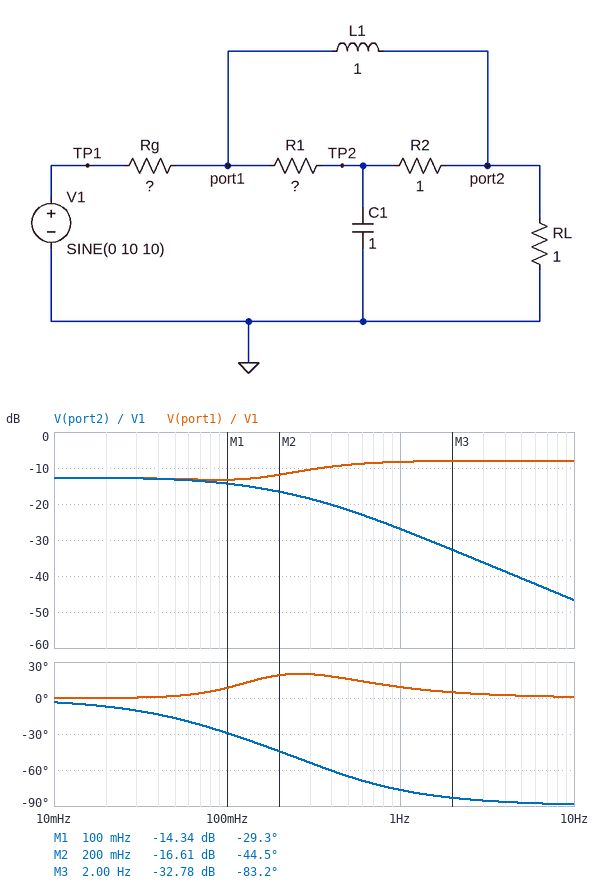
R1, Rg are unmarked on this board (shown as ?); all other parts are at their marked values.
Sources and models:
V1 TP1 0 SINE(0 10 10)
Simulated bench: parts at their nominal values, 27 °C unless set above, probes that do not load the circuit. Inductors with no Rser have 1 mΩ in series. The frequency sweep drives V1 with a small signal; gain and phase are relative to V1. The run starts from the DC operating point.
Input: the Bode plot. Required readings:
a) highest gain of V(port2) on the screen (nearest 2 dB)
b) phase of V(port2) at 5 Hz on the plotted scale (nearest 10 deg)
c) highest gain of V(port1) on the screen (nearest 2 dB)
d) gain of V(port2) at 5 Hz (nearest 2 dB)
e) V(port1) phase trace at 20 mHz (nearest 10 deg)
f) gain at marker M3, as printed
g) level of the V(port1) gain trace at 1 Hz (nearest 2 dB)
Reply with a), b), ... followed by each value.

a) -12 dB
b) -90 deg
c) -8 dB
d) -40 dB
e) 0 deg
f) -32.78 dB
g) -8 dB
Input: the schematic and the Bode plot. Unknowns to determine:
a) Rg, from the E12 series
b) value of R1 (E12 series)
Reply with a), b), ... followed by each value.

a) 3.3 Ω
b) 2.2 Ω
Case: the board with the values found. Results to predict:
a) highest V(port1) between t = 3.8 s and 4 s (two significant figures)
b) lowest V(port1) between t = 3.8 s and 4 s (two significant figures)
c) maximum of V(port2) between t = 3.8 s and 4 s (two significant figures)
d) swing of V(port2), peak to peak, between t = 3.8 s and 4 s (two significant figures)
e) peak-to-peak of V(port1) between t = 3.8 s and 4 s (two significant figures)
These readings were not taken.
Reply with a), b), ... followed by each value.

a) 4.0 V
b) -4.0 V
c) 47 mV
d) 93 mV
e) 8.0 V
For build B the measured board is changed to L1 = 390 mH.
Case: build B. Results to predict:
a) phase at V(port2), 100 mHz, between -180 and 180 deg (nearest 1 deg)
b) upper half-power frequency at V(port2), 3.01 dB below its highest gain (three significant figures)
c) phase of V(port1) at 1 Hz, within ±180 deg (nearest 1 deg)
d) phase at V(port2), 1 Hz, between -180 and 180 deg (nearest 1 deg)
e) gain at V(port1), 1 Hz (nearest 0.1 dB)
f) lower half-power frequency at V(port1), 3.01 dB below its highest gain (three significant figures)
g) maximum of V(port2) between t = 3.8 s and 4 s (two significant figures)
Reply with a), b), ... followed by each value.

a) -23 deg
b) 163 mHz
c) 22 deg
d) -58 deg
e) -9.8 dB
f) 709 mHz
g) 97 mV
